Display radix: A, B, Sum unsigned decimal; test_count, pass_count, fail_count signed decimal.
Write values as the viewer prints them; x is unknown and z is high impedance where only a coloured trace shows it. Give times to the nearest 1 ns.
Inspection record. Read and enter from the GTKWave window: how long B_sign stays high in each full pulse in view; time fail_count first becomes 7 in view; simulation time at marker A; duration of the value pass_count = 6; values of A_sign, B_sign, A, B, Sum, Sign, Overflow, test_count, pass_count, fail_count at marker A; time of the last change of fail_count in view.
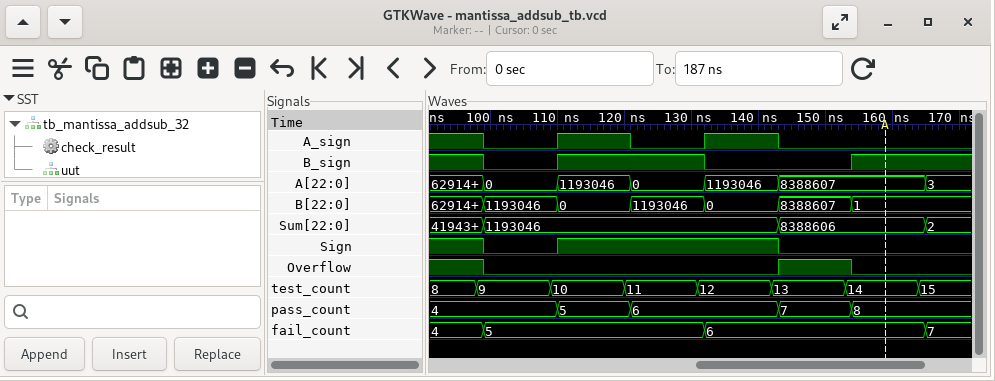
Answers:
22 ns
165 ns
159 ns
22 ns
A_sign=0, B_sign=1, A=8388607, B=1, Sum=8388606, Sign=0, Overflow=0, test_count=14, pass_count=8, fail_count=6
165 ns
